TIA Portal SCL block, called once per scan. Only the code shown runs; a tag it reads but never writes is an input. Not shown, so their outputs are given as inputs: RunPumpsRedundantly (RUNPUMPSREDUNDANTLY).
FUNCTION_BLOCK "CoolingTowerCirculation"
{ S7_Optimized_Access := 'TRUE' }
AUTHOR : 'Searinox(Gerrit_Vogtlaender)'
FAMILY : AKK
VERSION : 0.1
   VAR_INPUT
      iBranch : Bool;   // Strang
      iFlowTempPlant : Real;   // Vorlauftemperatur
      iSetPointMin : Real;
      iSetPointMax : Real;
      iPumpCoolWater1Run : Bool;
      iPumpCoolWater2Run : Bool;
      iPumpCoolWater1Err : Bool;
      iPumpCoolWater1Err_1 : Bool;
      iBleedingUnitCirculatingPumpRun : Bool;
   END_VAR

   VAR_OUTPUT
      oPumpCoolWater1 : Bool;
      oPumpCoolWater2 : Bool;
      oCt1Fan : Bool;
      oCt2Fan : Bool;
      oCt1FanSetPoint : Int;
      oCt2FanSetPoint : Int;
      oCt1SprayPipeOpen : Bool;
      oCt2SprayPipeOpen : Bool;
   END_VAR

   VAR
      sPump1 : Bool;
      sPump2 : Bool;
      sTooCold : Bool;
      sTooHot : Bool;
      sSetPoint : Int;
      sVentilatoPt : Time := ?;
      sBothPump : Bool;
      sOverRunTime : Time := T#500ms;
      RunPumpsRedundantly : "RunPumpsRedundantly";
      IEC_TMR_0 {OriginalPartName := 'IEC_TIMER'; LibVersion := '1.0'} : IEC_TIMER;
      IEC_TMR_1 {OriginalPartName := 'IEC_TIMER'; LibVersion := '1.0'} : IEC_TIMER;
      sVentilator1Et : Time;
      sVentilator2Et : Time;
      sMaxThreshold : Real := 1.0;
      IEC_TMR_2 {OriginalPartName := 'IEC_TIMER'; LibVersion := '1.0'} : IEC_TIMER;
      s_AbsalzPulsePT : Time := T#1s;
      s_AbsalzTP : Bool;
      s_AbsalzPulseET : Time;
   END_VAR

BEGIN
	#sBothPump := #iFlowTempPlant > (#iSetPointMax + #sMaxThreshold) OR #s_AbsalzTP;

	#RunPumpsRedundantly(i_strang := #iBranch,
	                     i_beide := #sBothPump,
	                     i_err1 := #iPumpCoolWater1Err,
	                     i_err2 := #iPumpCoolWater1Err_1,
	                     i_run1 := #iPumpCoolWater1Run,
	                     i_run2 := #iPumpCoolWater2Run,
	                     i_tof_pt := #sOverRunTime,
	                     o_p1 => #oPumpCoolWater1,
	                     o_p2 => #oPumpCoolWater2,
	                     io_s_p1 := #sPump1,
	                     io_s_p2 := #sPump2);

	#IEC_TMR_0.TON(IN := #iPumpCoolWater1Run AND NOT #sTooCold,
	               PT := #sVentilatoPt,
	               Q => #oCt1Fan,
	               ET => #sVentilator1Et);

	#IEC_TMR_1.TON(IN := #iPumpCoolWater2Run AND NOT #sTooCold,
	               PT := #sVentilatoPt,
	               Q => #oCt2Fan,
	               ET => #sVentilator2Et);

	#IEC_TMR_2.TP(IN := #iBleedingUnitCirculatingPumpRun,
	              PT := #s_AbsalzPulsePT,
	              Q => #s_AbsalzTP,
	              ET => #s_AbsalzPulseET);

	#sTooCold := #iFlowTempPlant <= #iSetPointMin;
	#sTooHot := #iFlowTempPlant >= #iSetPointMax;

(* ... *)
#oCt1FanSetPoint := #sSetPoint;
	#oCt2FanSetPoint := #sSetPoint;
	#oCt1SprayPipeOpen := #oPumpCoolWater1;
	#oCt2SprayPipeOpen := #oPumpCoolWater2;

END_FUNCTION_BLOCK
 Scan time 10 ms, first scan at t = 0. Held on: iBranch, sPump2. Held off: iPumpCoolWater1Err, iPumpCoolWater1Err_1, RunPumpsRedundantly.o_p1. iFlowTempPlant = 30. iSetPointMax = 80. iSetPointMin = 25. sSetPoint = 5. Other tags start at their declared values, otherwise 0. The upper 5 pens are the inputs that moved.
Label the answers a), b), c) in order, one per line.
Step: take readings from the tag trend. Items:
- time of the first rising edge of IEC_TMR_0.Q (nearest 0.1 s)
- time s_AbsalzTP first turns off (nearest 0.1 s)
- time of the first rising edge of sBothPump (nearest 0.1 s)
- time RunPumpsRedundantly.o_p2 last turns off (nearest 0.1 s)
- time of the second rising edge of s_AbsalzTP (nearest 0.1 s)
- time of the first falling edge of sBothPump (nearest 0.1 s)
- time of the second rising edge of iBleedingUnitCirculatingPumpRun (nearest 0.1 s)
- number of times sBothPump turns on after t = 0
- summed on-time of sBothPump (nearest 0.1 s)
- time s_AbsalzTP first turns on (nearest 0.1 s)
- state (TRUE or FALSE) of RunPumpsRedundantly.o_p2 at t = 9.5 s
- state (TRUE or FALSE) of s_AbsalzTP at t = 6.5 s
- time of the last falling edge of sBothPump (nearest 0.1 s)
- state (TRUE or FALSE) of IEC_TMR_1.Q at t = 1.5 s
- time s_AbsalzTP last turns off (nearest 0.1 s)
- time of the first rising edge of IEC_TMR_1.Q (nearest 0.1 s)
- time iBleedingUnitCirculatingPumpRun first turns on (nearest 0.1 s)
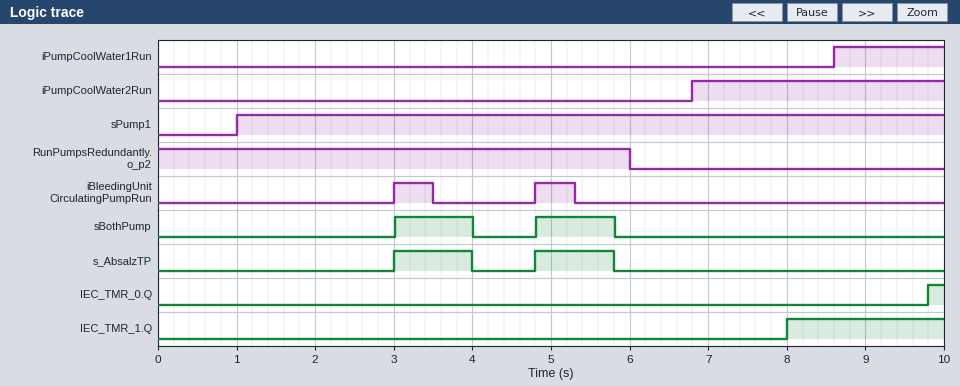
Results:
a) 9.8 s
b) 4.0 s
c) 3.0 s
d) 6.0 s
e) 4.8 s
f) 4.0 s
g) 4.8 s
h) 2
i) 2.0 s
j) 3.0 s
k) FALSE
l) FALSE
m) 5.8 s
n) FALSE
o) 5.8 s
p) 8.0 s
q) 3.0 s
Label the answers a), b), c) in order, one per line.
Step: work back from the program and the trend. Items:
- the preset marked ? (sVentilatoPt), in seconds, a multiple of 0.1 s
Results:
a) 1.2 s
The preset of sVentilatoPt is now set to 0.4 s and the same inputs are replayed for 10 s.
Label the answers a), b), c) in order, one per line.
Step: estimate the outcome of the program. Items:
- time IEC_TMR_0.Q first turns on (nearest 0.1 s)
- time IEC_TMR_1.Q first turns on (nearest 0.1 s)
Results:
a) 9.0 s
b) 7.2 s
